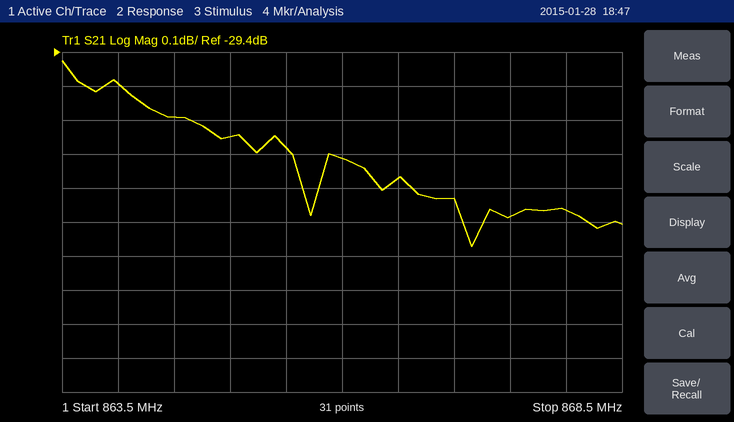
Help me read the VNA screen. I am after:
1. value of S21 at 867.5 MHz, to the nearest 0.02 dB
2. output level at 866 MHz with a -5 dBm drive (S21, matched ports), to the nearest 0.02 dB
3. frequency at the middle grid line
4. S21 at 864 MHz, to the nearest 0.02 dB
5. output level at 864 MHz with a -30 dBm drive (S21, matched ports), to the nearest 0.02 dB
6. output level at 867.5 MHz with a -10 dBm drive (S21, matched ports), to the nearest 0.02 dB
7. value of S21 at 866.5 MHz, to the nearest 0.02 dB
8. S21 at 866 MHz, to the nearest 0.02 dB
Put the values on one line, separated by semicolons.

-29.88 dB; -34.72 dBm; 866 MHz; -29.50 dB; -59.50 dBm; -39.88 dBm; -29.78 dB; -29.72 dB
